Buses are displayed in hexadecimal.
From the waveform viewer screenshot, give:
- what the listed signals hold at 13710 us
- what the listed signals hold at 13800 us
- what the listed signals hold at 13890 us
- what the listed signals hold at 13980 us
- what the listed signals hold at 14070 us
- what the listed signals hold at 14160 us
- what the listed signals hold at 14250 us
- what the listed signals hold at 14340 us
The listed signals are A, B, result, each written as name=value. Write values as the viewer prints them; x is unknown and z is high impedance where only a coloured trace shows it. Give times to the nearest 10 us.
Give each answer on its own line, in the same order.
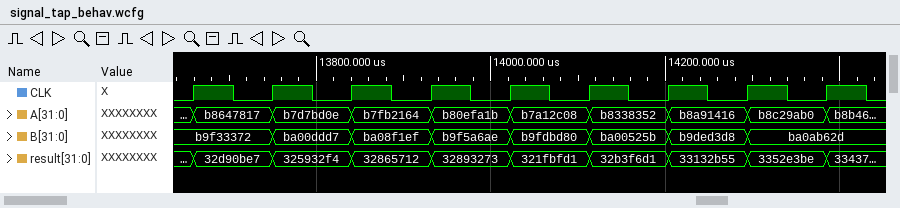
A=b8647817, B=b9f33372, result=32d90be7
A=b7d7bd0e, B=ba00ddd7, result=325932f4
A=b7fb2164, B=ba08f1ef, result=32865712
A=b80efa1b, B=b9f5a6ae, result=32893273
A=b7a12c08, B=b9fdbd80, result=321fbfd1
A=b8338352, B=ba00525b, result=32b3f6d1
A=b8a91416, B=b9ded3d8, result=33132b55
A=b8c29ab0, B=ba0ab62d, result=3352e3be
